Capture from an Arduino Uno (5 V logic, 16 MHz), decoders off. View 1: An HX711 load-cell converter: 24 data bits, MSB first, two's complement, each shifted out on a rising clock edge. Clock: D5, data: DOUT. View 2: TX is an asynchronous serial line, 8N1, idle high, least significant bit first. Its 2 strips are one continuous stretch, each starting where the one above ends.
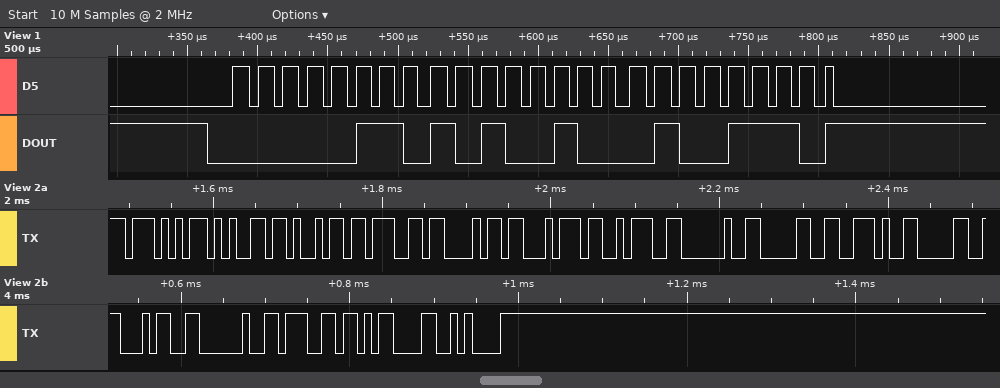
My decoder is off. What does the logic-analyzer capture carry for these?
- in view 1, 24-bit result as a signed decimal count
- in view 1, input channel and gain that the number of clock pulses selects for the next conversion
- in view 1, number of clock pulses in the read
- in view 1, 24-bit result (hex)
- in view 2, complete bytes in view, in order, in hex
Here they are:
435278
channel A, gain 128
25
0x06A44E
57 65 69 67 68 74 3A 20 30 2E 30 34 20 67 0D 0A
